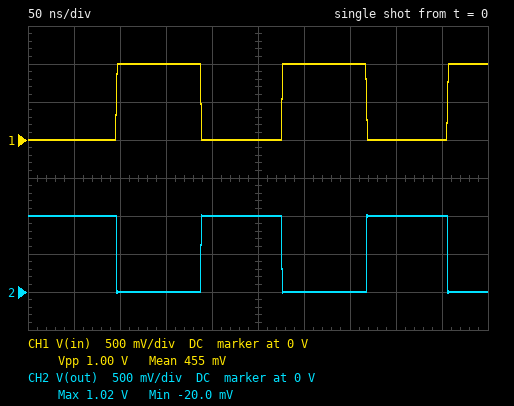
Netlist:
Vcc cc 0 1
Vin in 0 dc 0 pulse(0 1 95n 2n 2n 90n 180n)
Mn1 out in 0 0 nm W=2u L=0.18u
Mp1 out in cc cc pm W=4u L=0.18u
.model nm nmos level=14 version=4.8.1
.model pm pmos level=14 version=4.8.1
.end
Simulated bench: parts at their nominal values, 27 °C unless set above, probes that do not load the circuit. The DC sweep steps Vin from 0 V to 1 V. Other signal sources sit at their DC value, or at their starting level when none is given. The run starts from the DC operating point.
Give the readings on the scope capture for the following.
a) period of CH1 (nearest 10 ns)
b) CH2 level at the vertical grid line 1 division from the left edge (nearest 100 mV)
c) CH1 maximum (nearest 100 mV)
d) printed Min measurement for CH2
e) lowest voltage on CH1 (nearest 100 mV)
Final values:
180 ns
1.0 V
1.0 V
-20.0 mV
0 V
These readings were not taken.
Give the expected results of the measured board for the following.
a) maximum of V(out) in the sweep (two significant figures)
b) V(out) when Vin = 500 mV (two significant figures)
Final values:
1.0 V
460 mV
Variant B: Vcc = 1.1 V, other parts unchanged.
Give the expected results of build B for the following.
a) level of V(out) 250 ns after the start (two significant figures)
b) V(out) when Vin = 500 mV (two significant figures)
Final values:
1.1 V
970 mV
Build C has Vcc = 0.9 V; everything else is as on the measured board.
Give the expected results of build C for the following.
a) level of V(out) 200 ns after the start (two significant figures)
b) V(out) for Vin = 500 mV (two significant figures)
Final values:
900 mV
38 mV
